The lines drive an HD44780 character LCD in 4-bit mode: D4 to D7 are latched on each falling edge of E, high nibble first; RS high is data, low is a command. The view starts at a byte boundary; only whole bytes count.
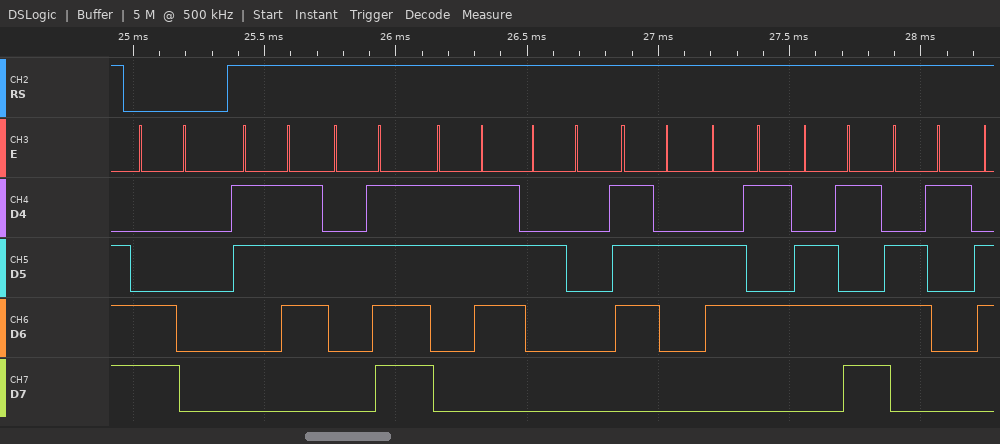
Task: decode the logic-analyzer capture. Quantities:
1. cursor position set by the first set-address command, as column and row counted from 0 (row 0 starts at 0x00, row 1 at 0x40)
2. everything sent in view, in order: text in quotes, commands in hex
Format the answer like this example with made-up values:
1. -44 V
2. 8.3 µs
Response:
1. column 0, row 1
2. 0xC0 "7/7 rema"
